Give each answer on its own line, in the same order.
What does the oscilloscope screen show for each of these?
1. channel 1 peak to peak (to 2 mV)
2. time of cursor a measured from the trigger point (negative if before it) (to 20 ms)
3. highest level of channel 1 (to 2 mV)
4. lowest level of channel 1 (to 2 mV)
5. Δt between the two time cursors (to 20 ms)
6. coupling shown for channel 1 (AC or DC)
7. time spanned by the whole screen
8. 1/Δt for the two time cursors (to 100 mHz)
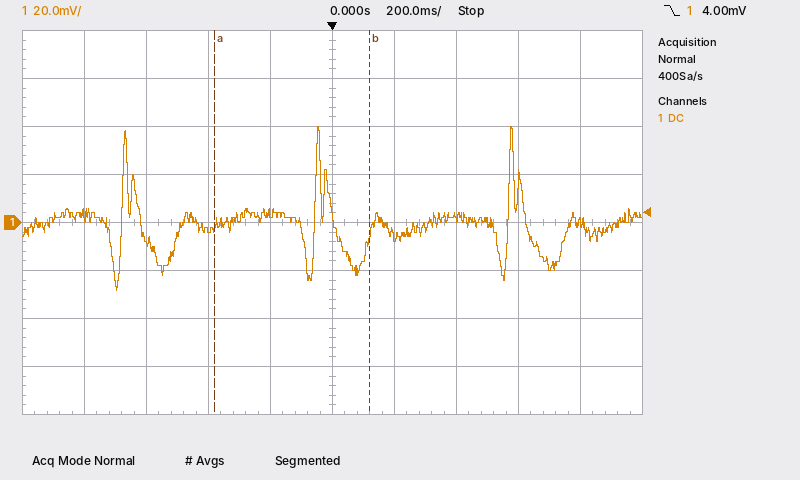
68 mV
-380 ms
40 mV
-28 mV
500 ms
DC
2 s
2.0 Hz
